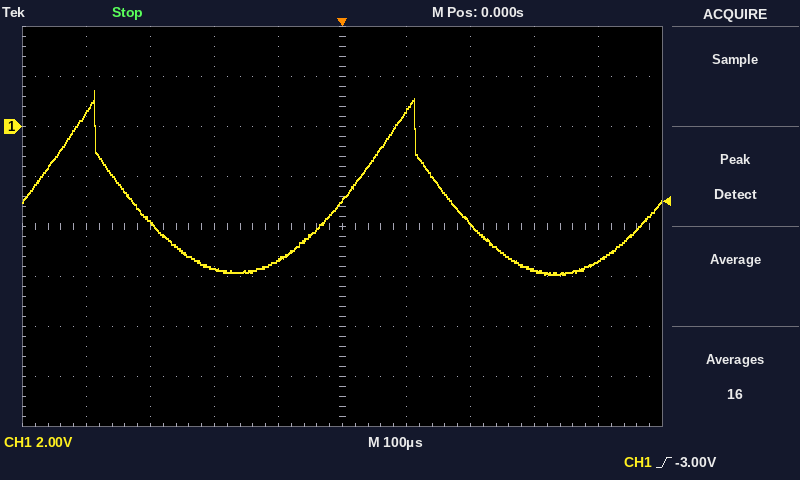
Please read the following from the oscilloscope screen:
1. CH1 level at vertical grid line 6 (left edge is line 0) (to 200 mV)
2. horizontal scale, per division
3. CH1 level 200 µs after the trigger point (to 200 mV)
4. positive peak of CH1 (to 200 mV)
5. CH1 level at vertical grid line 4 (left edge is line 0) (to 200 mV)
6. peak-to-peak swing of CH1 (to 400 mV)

600 mV
100 µs
-3.8 V
1.4 V
-5.4 V
7.2 V
